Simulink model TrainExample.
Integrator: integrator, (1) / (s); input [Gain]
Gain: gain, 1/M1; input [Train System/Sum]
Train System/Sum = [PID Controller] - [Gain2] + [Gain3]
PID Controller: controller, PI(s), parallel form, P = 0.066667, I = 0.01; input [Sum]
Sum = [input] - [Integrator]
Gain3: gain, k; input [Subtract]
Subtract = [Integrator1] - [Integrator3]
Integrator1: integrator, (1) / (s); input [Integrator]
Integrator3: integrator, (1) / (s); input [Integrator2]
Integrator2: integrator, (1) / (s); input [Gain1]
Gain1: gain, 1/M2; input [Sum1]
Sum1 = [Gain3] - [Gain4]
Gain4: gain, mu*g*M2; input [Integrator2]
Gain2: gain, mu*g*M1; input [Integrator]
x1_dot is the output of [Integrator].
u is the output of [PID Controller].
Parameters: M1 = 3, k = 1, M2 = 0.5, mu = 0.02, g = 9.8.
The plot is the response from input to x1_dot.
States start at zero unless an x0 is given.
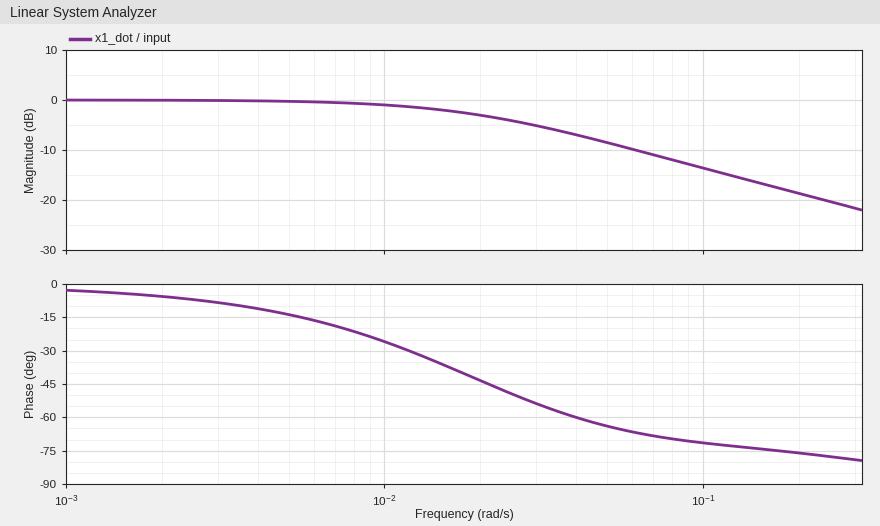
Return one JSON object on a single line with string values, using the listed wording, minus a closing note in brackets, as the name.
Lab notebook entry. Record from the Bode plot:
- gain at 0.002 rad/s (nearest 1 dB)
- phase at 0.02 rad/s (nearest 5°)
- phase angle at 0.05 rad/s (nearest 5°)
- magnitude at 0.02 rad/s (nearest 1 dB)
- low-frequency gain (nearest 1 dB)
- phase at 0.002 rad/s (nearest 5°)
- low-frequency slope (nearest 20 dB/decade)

{"gain at 0.002 rad/s": "0 dB", "phase at 0.02 rad/s": "-45°", "phase angle at 0.05 rad/s": "-65°", "magnitude at 0.02 rad/s": "-3 dB", "low-frequency gain": "0 dB", "phase at 0.002 rad/s": "-5°", "low-frequency slope": "0 dB/decade"}
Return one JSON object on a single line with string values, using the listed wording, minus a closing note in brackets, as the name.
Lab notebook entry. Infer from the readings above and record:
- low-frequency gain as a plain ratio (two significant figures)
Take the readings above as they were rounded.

{"low-frequency gain as a plain ratio": "1.0"}
